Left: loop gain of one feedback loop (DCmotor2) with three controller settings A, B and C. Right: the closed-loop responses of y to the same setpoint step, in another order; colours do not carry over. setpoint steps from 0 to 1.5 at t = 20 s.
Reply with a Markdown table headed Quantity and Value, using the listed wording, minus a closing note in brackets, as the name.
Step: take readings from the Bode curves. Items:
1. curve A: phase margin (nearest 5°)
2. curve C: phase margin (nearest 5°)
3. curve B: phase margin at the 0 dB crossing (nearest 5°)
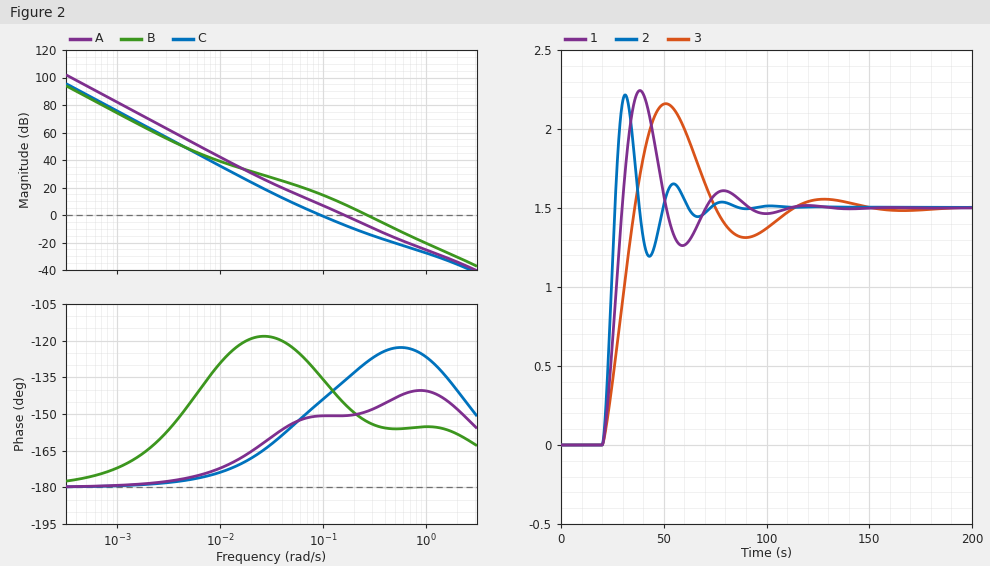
| Quantity | Value |
|---|---|
| curve A: phase margin | 30° |
| curve C: phase margin | 35° |
| curve B: phase margin at the 0 dB crossing | 25° |
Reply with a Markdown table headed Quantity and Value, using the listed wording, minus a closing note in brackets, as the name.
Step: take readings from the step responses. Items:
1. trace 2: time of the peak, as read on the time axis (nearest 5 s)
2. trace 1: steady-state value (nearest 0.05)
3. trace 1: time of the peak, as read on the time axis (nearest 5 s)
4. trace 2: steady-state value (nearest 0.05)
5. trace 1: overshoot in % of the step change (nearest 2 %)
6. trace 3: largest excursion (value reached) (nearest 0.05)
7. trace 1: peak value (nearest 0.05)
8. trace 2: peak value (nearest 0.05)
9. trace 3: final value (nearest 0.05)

| Quantity | Value |
|---|---|
| trace 2: time of the peak, as read on the time axis | 30 s |
| trace 1: steady-state value | 1.50 |
| trace 1: time of the peak, as read on the time axis | 40 s |
| trace 2: steady-state value | 1.50 |
| trace 1: overshoot in % of the step change | 50 % |
| trace 3: largest excursion (value reached) | 2.15 |
| trace 1: peak value | 2.25 |
| trace 2: peak value | 2.20 |
| trace 3: final value | 1.50 |
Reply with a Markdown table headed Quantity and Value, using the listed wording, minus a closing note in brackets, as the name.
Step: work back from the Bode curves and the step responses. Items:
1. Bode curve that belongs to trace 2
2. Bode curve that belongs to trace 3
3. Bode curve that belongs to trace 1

| Quantity | Value |
|---|---|
| Bode curve that belongs to trace 2 | B |
| Bode curve that belongs to trace 3 | C |
| Bode curve that belongs to trace 1 | A |
